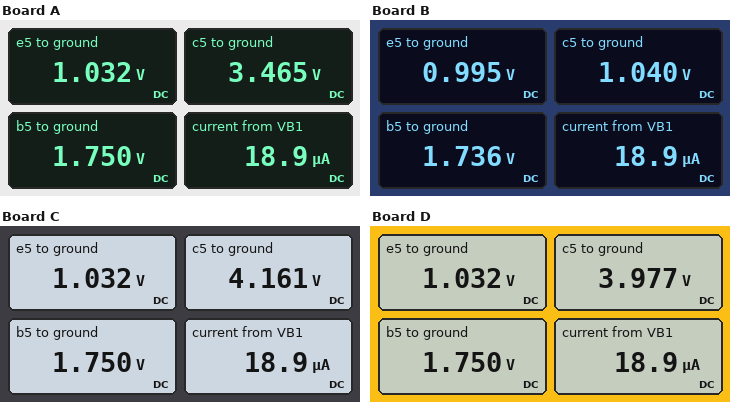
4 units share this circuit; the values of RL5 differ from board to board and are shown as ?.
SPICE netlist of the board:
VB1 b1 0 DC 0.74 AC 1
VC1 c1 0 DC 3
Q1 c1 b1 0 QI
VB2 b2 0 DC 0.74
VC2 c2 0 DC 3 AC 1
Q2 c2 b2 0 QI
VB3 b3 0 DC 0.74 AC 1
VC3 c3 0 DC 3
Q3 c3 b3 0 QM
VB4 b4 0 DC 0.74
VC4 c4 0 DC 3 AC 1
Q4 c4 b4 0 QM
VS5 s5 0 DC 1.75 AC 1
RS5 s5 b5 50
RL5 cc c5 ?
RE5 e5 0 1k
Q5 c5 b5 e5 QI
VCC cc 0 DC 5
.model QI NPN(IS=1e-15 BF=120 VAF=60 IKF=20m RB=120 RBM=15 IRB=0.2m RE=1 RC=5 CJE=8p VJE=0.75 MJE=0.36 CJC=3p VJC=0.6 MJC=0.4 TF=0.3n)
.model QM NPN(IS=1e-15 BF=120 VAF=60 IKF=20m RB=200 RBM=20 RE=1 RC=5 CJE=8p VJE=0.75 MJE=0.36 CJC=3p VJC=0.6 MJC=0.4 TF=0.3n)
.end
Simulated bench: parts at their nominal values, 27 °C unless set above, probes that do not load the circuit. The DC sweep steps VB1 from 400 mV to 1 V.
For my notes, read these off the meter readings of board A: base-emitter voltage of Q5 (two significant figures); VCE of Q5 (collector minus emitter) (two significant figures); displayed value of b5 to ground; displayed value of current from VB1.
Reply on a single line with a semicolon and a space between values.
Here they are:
720 mV; 2.4 V; 1.750 V; 18.9 µA
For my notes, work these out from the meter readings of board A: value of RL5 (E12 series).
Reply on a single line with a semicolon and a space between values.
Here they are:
1.5 kΩ
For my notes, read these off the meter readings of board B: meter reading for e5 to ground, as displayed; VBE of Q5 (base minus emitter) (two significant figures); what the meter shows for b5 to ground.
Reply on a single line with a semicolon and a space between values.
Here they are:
0.995 V; 740 mV; 1.736 V
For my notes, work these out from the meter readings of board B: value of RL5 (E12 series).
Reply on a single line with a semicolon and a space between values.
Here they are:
5.6 kΩ
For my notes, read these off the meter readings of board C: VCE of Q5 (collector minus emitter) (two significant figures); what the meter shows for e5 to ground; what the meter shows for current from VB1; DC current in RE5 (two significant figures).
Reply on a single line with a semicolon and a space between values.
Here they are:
3.1 V; 1.032 V; 18.9 µA; 1.0 mA
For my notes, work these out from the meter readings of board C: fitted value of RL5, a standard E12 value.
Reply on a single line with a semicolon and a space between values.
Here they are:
820 Ω
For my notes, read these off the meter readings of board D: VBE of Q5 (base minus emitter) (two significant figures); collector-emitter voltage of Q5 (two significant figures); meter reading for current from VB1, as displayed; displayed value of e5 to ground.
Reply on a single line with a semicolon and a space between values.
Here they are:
720 mV; 2.9 V; 18.9 µA; 1.032 V
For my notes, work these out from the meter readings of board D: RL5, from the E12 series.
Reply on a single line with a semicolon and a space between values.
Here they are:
1 kΩ
